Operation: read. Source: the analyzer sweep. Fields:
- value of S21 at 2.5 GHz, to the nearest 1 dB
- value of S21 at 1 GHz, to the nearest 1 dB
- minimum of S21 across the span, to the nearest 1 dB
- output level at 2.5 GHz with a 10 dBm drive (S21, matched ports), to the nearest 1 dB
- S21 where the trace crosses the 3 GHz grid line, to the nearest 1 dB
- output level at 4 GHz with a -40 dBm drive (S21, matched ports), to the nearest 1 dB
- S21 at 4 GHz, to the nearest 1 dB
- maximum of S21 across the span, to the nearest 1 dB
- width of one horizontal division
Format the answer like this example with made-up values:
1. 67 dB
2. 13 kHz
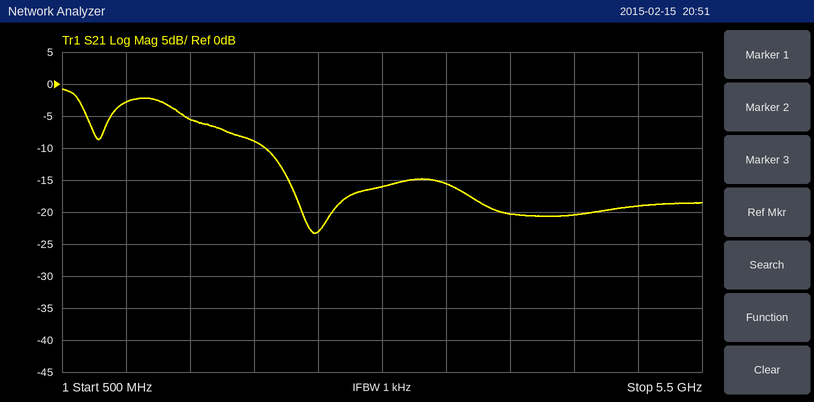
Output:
1. -23 dB
2. -3 dB
3. -23 dB
4. -13 dBm
5. -16 dB
6. -60 dBm
7. -20 dB
8. -1 dB
9. 500 MHz
